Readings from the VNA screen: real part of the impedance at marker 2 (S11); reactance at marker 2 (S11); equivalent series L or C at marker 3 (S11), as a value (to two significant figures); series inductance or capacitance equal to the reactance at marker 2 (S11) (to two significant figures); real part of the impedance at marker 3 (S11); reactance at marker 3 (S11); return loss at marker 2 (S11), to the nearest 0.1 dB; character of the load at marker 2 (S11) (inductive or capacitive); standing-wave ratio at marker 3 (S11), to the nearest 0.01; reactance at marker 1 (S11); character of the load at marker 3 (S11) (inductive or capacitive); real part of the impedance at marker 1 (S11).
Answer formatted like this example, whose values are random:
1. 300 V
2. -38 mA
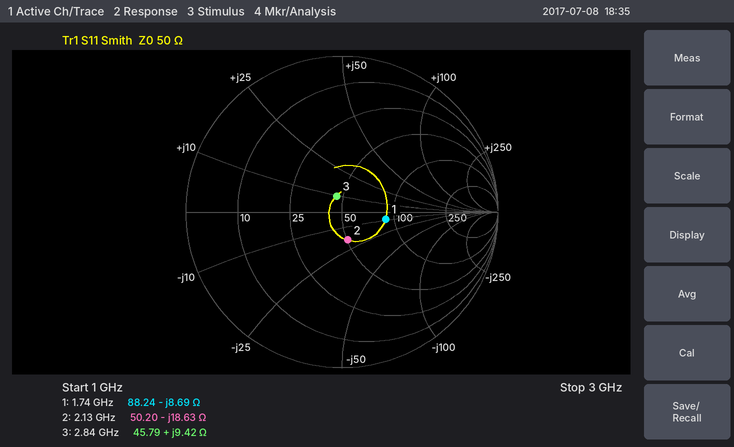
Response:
1. 50.20 Ω
2. -18.63 Ω
3. 530 pH
4. 4.0 pF
5. 45.79 Ω
6. +9.42 Ω
7. 14.8 dB
8. capacitive
9. 1.24
10. -8.69 Ω
11. inductive
12. 88.24 Ω
